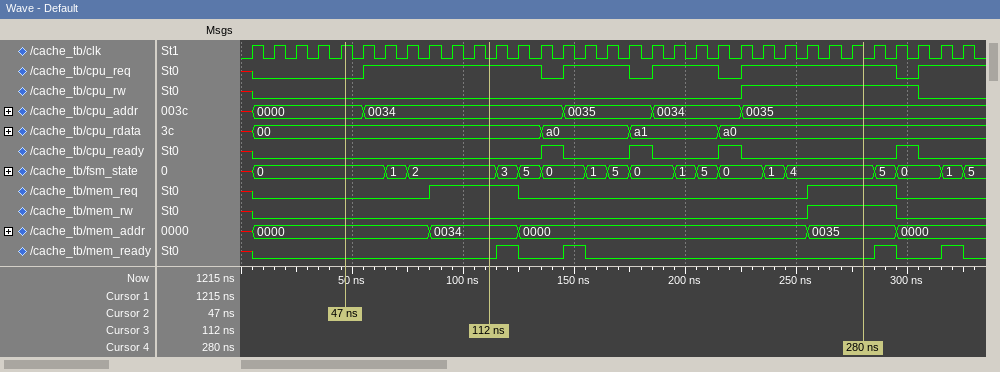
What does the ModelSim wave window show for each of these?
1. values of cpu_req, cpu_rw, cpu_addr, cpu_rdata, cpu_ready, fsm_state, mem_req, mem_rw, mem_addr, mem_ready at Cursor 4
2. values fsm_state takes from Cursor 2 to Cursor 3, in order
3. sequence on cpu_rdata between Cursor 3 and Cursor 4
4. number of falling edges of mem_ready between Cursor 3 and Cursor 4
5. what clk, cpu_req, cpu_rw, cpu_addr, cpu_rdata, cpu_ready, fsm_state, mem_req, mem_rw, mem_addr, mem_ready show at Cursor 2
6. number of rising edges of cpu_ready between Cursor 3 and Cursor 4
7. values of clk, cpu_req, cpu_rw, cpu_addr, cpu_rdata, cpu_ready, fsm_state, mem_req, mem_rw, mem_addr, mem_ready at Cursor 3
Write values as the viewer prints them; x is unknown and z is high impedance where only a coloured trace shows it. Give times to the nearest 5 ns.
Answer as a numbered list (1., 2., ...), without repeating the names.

1. cpu_req=1, cpu_rw=1, cpu_addr=0035, cpu_rdata=a0, cpu_ready=0, fsm_state=4, mem_req=1, mem_rw=1, mem_addr=0035, mem_ready=0
2. 0, 1, 2
3. 00, a0, a1, a0
4. 2
5. clk=1, cpu_req=0, cpu_rw=0, cpu_addr=0000, cpu_rdata=00, cpu_ready=0, fsm_state=0, mem_req=0, mem_rw=0, mem_addr=0000, mem_ready=0
6. 3
7. clk=0, cpu_req=1, cpu_rw=0, cpu_addr=0034, cpu_rdata=00, cpu_ready=0, fsm_state=2, mem_req=1, mem_rw=0, mem_addr=0034, mem_ready=0
